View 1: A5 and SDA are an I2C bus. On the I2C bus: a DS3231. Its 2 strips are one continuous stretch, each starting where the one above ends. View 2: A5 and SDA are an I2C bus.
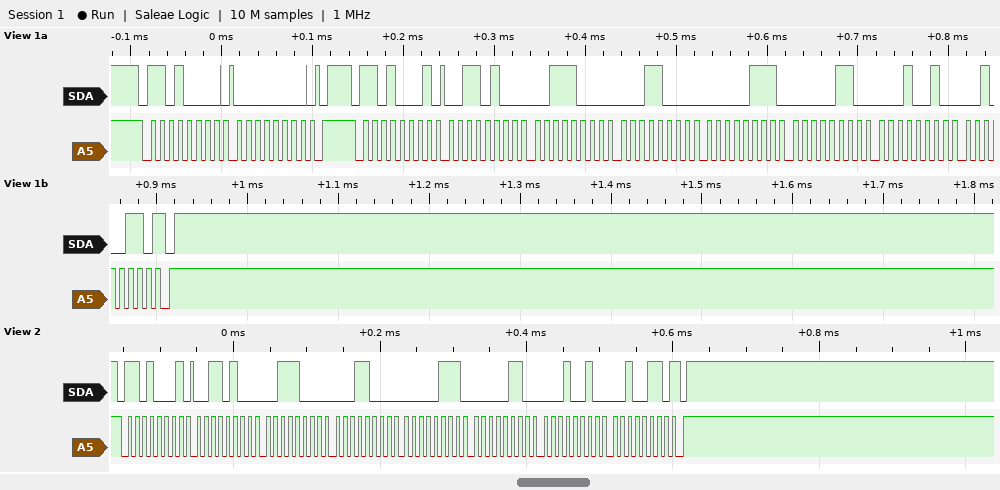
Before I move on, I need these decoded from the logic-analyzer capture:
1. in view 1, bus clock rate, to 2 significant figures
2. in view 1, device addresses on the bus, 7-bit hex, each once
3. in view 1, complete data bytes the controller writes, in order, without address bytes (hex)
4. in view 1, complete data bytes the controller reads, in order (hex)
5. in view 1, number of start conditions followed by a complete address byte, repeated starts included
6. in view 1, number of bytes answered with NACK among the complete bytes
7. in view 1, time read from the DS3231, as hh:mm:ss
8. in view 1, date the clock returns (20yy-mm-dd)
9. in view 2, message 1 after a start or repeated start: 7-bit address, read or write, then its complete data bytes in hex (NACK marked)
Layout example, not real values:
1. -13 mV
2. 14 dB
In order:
1. 100 kHz
2. 0x68
3. 00
4. 34 38 18 07 06 12 26
5. 2
6. 1
7. 18:38:34
8. 2026-12-06
9. 0x68 read: 34 38 18 07 06 12 26 NACK
